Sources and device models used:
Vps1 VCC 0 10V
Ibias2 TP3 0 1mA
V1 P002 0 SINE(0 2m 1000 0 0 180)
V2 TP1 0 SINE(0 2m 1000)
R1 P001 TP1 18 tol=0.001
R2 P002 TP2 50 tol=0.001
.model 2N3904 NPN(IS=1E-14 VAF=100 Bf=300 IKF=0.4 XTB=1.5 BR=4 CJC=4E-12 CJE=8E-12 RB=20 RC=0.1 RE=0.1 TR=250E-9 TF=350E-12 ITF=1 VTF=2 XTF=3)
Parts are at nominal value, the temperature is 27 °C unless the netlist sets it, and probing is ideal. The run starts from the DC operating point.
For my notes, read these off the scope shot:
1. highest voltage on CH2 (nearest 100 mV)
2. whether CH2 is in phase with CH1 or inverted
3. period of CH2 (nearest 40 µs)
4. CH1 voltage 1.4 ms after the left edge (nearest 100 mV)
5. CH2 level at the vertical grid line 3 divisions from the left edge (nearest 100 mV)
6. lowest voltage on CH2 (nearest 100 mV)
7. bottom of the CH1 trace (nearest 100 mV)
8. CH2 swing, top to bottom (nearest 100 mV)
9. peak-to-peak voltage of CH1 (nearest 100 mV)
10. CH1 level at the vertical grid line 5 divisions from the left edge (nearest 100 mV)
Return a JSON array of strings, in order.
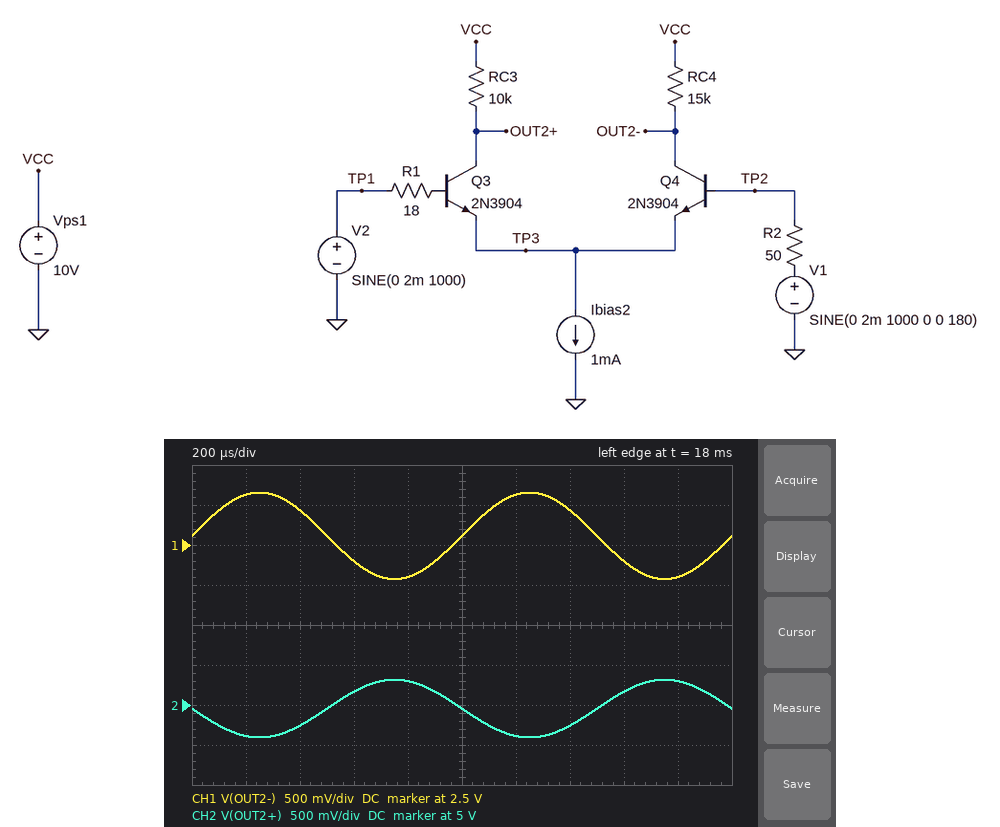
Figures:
["5.3 V", "inverted", "1.00 ms", "2.9 V", "5.2 V", "4.6 V", "2.1 V", "700 mV", "1.1 V", "2.6 V"]
